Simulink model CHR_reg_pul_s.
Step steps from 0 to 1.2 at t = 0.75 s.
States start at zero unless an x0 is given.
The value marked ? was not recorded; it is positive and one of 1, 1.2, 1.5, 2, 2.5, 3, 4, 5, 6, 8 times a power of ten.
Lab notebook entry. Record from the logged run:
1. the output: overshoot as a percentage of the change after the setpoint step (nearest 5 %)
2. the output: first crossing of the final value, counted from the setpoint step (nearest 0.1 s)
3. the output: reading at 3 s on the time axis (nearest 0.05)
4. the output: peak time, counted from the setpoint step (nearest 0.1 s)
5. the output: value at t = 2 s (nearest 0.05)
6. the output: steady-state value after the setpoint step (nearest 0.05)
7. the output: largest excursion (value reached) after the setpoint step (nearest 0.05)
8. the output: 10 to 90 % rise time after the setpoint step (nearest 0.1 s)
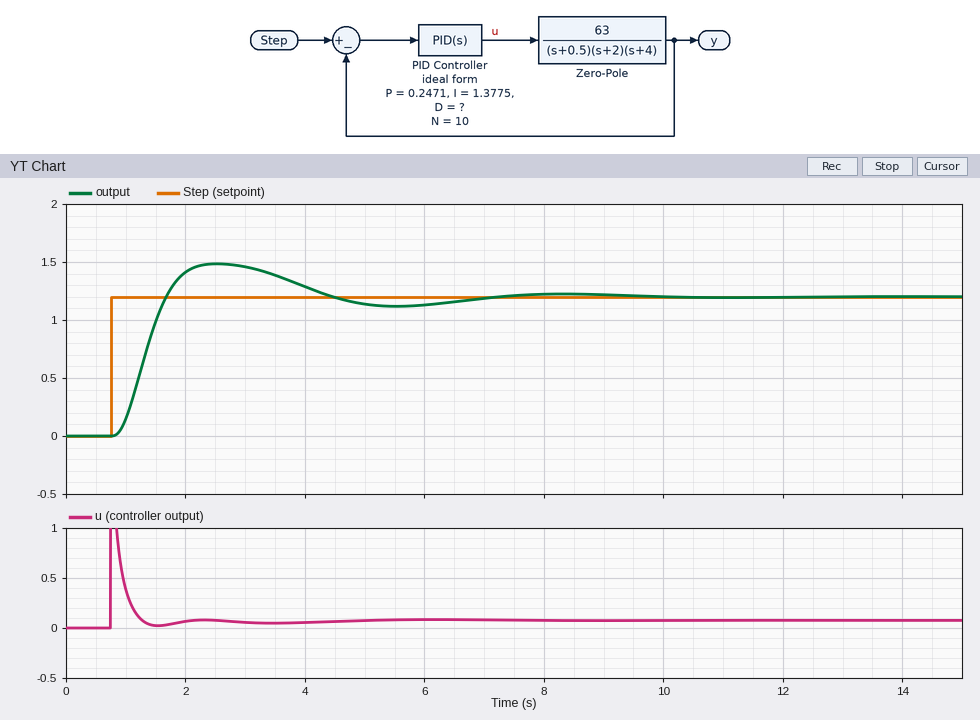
25 %
0.9 s
1.45
1.8 s
1.40
1.20
1.50
0.6 s
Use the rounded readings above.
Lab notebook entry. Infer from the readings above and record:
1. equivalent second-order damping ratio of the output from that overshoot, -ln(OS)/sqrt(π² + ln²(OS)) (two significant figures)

0.40
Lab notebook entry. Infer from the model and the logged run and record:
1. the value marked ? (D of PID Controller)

0.6
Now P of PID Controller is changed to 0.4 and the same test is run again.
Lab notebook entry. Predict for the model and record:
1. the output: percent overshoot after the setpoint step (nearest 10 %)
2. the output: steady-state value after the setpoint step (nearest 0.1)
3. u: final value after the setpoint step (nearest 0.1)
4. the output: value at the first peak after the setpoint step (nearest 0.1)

30 %
1.2
0.1
1.6
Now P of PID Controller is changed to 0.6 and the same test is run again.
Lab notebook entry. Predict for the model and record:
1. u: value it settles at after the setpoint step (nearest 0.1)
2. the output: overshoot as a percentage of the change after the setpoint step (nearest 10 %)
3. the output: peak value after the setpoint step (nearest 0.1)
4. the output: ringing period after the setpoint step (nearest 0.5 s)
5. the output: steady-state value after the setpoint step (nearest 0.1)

0.1
40 %
1.7
1.5 s
1.2
